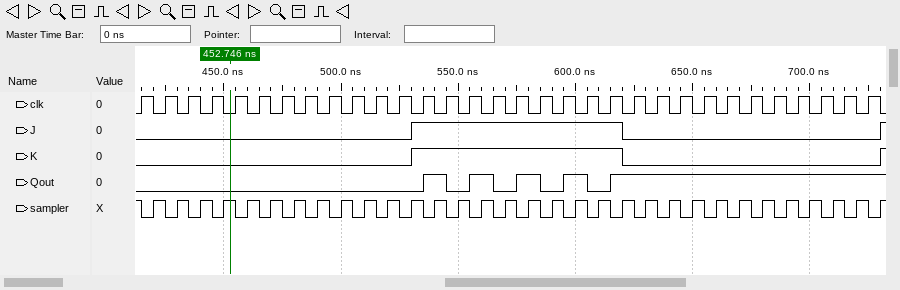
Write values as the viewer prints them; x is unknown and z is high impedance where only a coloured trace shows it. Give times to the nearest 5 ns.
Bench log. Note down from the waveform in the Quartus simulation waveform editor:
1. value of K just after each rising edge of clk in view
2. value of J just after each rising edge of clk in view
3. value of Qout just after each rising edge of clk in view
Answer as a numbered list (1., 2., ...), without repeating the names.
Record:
1. 0 0 0 0 0 0 0 0 0 0 0 0 1 1 1 1 1 1 1 1 1 0 0 0 0 0 0 0 0 0 0 0
2. 0 0 0 0 0 0 0 0 0 0 0 0 1 1 1 1 1 1 1 1 1 0 0 0 0 0 0 0 0 0 0 0
3. 0 0 0 0 0 0 0 0 0 0 0 0 1 0 1 0 1 0 1 0 1 1 1 1 1 1 1 1 1 1 1 1
